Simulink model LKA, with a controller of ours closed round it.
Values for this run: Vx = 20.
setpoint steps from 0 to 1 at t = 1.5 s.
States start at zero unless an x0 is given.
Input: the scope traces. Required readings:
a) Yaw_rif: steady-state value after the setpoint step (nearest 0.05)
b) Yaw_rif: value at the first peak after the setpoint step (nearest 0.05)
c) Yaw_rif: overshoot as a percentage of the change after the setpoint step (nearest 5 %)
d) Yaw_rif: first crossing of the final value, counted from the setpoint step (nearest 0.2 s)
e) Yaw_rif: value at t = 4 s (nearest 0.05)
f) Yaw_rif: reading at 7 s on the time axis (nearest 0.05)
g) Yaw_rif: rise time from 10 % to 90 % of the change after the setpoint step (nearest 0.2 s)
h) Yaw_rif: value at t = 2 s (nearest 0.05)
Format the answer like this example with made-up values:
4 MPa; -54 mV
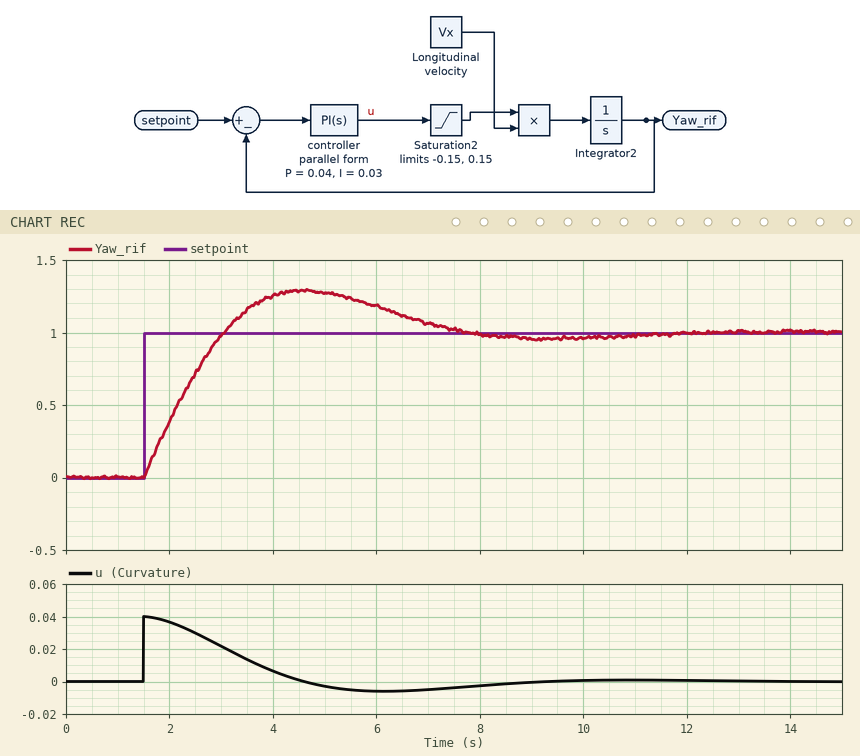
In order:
1.00; 1.30; 30 %; 1.6 s; 1.25; 1.05; 1.2 s; 0.40
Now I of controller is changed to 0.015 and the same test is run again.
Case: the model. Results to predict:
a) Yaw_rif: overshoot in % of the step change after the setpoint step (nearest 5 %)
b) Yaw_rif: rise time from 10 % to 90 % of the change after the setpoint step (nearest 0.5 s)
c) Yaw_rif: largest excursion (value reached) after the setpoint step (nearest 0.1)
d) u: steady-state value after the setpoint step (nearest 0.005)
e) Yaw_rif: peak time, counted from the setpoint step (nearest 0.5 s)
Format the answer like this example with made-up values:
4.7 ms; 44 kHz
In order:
20 %; 1.5 s; 1.2; 0.000; 4.0 s
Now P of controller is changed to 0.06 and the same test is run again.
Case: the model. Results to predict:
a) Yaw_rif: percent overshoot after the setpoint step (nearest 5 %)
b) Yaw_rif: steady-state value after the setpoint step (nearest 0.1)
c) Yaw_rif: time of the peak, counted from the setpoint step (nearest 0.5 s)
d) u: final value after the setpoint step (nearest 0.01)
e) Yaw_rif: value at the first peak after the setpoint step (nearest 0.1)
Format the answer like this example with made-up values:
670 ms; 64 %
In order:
20 %; 1.0; 3.0 s; 0.00; 1.2
